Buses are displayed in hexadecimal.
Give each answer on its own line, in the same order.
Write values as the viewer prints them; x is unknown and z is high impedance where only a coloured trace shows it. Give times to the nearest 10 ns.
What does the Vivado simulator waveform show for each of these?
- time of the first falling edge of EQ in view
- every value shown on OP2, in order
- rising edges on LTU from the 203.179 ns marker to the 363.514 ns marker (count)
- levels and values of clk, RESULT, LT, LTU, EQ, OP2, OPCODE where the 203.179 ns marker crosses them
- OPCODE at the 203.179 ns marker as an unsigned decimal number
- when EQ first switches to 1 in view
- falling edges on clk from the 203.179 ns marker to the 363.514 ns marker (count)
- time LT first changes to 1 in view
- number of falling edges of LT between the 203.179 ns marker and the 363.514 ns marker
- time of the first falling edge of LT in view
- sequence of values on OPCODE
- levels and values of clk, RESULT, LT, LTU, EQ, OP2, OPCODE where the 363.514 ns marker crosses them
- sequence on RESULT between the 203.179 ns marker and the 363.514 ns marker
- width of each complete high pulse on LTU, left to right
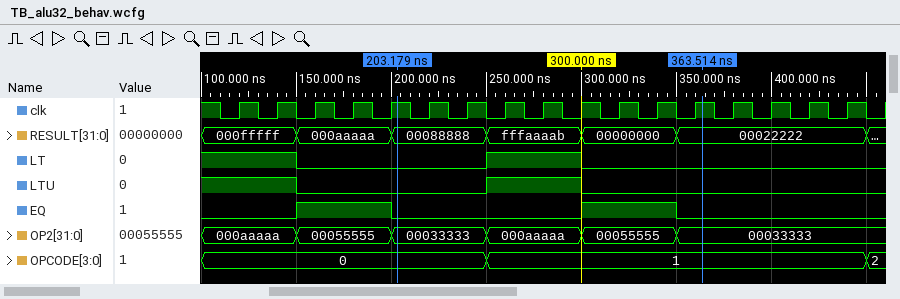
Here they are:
200 ns
000aaaaa, 00055555, 00033333, 000aaaaa, 00055555, 00033333
1
clk=1, RESULT=00088888, LT=0, LTU=0, EQ=0, OP2=00033333, OPCODE=0
0
150 ns
8
250 ns
1
150 ns
0, 1, 2
clk=1, RESULT=00022222, LT=0, LTU=0, EQ=0, OP2=00033333, OPCODE=1
00088888, fffaaaab, 00000000, 00022222
50 ns
